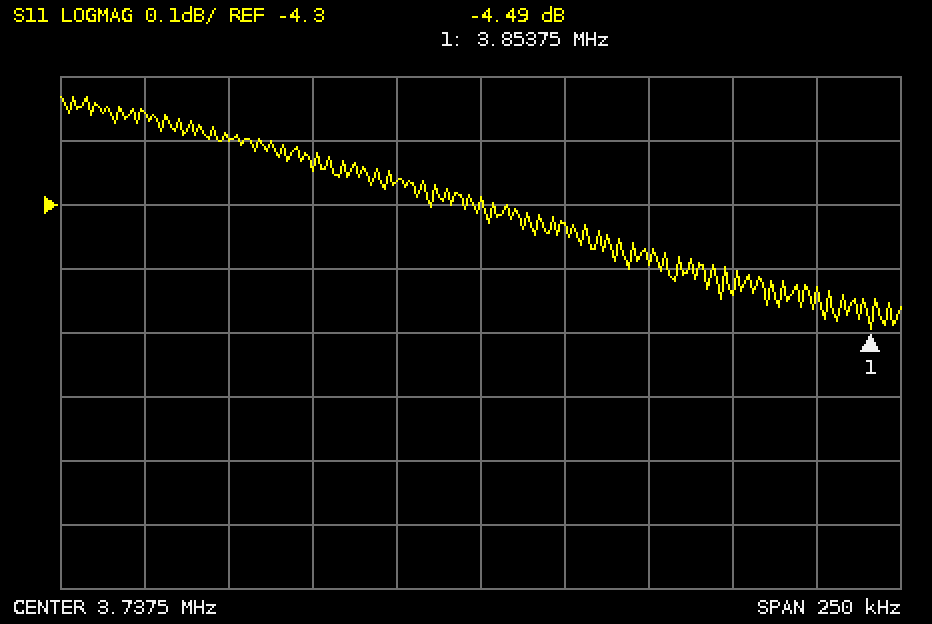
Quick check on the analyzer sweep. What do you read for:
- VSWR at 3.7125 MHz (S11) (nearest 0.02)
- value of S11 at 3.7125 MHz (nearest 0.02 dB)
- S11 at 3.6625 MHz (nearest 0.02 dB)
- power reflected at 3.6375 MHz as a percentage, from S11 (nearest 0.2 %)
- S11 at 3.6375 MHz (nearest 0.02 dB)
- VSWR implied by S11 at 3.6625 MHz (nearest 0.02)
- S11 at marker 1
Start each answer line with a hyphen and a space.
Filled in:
- 4.16
- -4.26 dB
- -4.20 dB
- 38.4 %
- -4.16 dB
- 4.22
- -4.49 dB
